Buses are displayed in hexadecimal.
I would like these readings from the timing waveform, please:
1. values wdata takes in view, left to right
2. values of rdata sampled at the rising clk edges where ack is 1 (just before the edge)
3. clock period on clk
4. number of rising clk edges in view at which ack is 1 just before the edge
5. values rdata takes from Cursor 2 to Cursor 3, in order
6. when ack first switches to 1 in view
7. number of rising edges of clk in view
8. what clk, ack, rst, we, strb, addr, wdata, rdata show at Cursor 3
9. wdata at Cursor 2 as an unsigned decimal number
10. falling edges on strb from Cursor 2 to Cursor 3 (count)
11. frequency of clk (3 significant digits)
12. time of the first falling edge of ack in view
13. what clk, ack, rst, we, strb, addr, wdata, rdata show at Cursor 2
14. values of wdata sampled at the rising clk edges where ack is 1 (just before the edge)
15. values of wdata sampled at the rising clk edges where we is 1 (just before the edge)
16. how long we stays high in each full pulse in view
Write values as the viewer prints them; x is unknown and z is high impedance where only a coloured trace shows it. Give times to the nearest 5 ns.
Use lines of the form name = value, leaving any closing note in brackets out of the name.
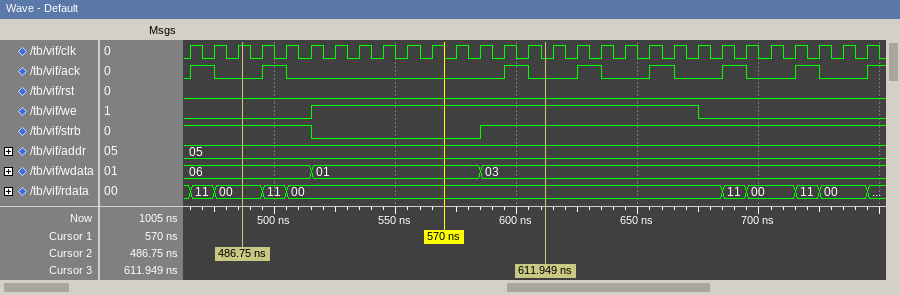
values wdata takes in view, left to right = 06, 01, 03
values of rdata sampled at the rising clk edges where ack is 1 = 11, 11, 00, 00, 00, 11, 11
clock period on clk = 10 ns
number of rising clk edges in view at which ack is 1 just before the edge = 7
values rdata takes from Cursor 2 to Cursor 3, in order = 00, 11, 00
when ack first switches to 1 in view = 465 ns
number of rising edges of clk in view = 29
what clk, ack, rst, we, strb, addr, wdata, rdata show at Cursor 3 = clk=0, ack=0, rst=0, we=1, strb=1, addr=05, wdata=03, rdata=00
wdata at Cursor 2 as an unsigned decimal number = 6
falling edges on strb from Cursor 2 to Cursor 3 = 1
frequency of clk = 100 MHz
time of the first falling edge of ack in view = 475 ns
what clk, ack, rst, we, strb, addr, wdata, rdata show at Cursor 2 = clk=1, ack=0, rst=0, we=0, strb=1, addr=05, wdata=06, rdata=00
values of wdata sampled at the rising clk edges where ack is 1 = 06, 06, 03, 03, 03, 03, 03
values of wdata sampled at the rising clk edges where we is 1 = 01, 01, 01, 01, 01, 01, 01, 03, 03, 03, 03, 03, 03, 03, 03, 03
how long we stays high in each full pulse in view = 160 ns
